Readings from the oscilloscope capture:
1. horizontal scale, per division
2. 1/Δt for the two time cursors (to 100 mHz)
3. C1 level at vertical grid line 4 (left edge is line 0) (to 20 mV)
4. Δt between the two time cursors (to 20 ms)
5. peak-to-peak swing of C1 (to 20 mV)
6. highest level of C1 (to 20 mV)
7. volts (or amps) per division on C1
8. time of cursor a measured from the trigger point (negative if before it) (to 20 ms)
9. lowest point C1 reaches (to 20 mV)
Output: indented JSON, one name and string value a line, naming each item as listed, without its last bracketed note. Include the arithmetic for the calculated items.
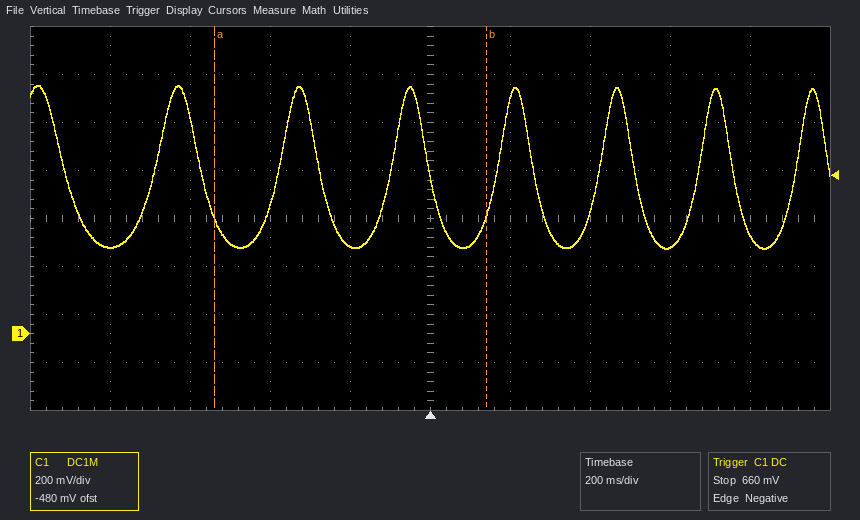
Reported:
{
  "horizontal scale, per division": "200 ms",
  "1/Δt for the two time cursors": "1 / 680 ms ≈ 1.5 Hz",
  "C1 level at vertical grid line 4 (left edge is line 0)": "360 mV",
  "Δt between the two time cursors": "680 ms",
  "peak-to-peak swing of C1": "1.04 V − (360 mV) = 680 mV",
  "highest level of C1": "1.04 V",
  "volts (or amps) per division on C1": "200 mV",
  "time of cursor a measured from the trigger point (negative if before it)": "-540 ms",
  "lowest point C1 reaches": "360 mV"
}
